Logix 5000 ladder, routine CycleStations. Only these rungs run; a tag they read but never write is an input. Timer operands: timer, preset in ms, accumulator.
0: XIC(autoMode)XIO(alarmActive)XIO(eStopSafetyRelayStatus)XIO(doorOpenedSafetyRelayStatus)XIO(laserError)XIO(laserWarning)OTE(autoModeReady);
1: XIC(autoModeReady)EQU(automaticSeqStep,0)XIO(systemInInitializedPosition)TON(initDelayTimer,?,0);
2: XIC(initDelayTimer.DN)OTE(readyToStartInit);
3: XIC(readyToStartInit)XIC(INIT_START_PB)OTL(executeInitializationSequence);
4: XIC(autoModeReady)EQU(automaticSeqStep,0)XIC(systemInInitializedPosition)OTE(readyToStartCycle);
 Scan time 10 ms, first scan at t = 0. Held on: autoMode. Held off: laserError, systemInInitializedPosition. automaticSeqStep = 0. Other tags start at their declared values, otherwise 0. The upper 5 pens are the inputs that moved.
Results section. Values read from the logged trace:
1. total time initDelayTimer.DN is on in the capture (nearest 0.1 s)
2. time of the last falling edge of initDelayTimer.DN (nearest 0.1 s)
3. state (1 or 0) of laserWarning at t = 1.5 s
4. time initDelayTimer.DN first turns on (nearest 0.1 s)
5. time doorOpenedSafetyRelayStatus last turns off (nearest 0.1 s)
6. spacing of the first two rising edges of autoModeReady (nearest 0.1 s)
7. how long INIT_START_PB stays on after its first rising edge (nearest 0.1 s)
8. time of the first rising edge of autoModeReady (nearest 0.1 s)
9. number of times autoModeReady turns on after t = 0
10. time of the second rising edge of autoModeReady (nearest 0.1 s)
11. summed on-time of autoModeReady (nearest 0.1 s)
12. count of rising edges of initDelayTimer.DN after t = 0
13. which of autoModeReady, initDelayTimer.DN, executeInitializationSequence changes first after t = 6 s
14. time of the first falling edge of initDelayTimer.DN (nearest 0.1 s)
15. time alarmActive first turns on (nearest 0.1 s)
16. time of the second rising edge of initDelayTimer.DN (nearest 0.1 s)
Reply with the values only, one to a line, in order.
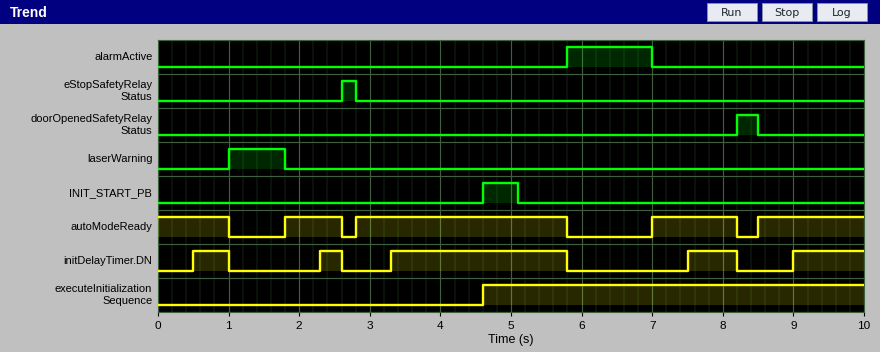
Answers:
5.0 s
8.2 s
1
0.5 s
8.5 s
1.0 s
0.5 s
1.8 s
4
2.8 s
7.5 s
5
autoModeReady
1.0 s
5.8 s
2.3 s
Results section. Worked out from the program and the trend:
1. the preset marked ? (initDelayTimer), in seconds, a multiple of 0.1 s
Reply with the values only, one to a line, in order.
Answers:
0.5 s
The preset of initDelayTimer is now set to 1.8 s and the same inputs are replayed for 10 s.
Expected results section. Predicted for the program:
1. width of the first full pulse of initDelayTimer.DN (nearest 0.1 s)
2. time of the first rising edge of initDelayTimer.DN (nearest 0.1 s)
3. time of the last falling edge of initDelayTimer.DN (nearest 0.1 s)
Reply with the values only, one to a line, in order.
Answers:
1.2 s
4.6 s
5.8 s
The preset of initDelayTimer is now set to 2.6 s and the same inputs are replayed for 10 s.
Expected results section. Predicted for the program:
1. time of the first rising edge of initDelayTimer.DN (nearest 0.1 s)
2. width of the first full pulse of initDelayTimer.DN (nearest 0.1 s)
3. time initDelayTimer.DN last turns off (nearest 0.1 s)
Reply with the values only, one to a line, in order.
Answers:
5.4 s
0.4 s
5.8 s
